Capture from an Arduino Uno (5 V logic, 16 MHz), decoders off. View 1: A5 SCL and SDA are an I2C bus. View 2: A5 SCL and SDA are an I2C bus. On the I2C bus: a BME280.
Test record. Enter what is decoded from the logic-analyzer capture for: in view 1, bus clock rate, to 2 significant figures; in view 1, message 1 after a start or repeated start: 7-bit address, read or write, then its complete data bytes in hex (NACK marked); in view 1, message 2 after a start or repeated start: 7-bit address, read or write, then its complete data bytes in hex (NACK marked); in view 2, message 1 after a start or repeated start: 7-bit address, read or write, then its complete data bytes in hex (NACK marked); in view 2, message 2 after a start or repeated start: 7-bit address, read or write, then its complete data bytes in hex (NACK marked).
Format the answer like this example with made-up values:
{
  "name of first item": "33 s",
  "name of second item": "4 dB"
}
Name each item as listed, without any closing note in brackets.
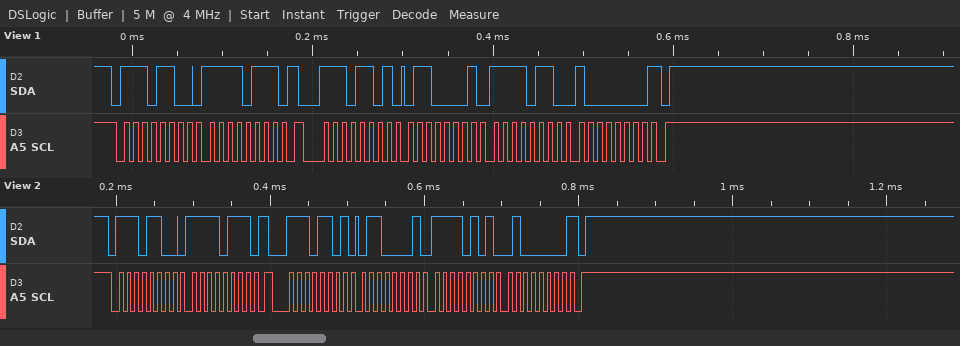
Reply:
{
  "in view 1, bus clock rate, to 2 significant figures": "100 kHz",
  "in view 1, message 1 after a start or repeated start: 7-bit address, read or write, then its complete data bytes in hex": "0x76 write: F7",
  "in view 1, message 2 after a start or repeated start: 7-bit address, read or write, then its complete data bytes in hex": "0x76 read: 61 F6 80 NACK",
  "in view 2, message 1 after a start or repeated start: 7-bit address, read or write, then its complete data bytes in hex": "0x76 write: F7",
  "in view 2, message 2 after a start or repeated start: 7-bit address, read or write, then its complete data bytes in hex": "0x76 read: 61 F5 40 NACK"
}
